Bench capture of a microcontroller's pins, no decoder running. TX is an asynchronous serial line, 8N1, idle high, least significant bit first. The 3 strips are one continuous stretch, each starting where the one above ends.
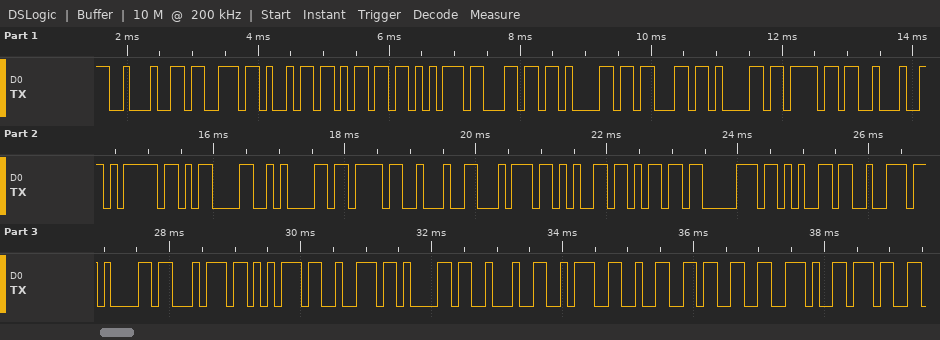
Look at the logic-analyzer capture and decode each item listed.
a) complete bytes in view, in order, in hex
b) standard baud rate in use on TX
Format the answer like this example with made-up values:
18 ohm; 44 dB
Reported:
0x22 0x73 0x69 0x6D 0x75 0x6C 0x61 0x63 0x61 0x6F 0x22 0x7D 0x0D 0x0A 0x7B 0x22 0x74 0x65 0x6D 0x70 0x65 0x72 0x61 0x74 0x75 0x72 0x61 0x22 0x3A 0x32 0x33 0x2E 0x37; 9600 baud
